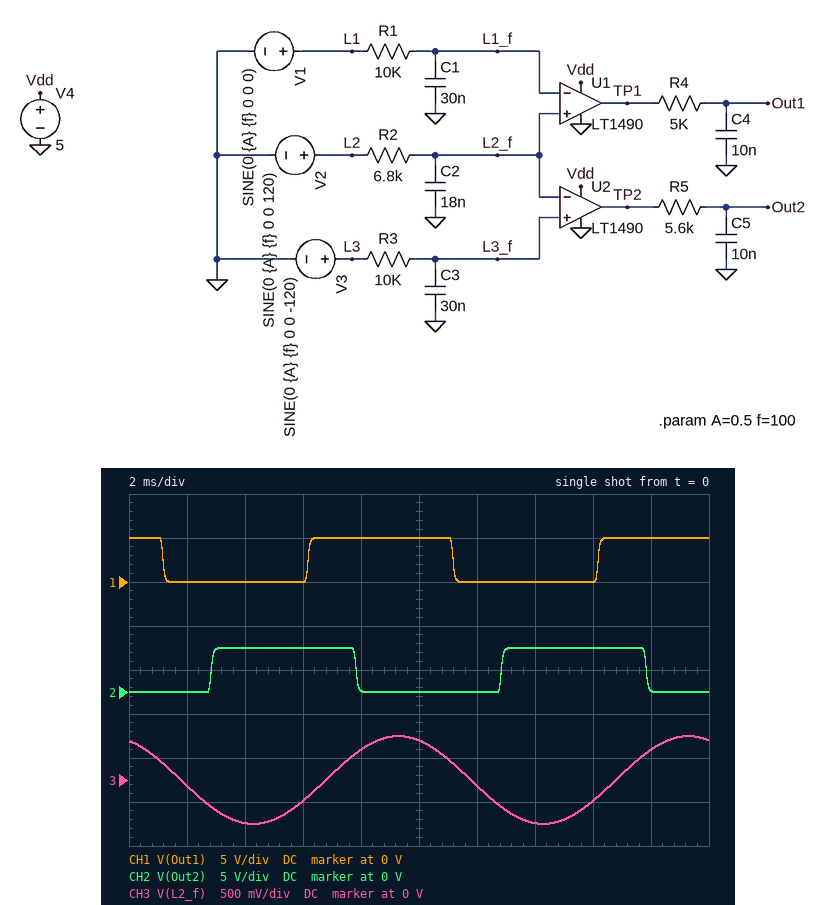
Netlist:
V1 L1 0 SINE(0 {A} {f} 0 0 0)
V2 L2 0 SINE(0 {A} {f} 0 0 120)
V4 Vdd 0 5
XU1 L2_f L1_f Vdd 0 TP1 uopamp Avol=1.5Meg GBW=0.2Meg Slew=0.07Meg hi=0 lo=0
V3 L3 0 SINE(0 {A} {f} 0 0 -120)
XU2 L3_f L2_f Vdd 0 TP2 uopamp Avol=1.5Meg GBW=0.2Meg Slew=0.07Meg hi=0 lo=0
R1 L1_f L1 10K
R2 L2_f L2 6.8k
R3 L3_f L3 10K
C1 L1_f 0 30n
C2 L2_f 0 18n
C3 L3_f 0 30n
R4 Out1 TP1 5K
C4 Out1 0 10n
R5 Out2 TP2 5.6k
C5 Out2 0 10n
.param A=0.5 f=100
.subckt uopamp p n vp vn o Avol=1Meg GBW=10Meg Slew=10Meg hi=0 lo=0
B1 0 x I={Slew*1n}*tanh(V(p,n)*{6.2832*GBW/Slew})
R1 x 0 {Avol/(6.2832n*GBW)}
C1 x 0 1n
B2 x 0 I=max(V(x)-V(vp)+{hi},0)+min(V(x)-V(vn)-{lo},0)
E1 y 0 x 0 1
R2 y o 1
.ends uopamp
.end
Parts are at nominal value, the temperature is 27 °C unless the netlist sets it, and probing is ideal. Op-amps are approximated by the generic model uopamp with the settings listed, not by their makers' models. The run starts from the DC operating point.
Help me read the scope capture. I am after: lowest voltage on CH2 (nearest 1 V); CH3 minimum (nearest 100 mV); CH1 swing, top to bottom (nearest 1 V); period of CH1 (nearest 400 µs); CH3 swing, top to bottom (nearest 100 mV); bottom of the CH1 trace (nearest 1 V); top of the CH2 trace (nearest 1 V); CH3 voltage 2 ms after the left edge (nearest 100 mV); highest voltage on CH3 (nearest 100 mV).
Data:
0 V
-500 mV
5 V
10.0 ms
1.0 V
0 V
5 V
-100 mV
500 mV
